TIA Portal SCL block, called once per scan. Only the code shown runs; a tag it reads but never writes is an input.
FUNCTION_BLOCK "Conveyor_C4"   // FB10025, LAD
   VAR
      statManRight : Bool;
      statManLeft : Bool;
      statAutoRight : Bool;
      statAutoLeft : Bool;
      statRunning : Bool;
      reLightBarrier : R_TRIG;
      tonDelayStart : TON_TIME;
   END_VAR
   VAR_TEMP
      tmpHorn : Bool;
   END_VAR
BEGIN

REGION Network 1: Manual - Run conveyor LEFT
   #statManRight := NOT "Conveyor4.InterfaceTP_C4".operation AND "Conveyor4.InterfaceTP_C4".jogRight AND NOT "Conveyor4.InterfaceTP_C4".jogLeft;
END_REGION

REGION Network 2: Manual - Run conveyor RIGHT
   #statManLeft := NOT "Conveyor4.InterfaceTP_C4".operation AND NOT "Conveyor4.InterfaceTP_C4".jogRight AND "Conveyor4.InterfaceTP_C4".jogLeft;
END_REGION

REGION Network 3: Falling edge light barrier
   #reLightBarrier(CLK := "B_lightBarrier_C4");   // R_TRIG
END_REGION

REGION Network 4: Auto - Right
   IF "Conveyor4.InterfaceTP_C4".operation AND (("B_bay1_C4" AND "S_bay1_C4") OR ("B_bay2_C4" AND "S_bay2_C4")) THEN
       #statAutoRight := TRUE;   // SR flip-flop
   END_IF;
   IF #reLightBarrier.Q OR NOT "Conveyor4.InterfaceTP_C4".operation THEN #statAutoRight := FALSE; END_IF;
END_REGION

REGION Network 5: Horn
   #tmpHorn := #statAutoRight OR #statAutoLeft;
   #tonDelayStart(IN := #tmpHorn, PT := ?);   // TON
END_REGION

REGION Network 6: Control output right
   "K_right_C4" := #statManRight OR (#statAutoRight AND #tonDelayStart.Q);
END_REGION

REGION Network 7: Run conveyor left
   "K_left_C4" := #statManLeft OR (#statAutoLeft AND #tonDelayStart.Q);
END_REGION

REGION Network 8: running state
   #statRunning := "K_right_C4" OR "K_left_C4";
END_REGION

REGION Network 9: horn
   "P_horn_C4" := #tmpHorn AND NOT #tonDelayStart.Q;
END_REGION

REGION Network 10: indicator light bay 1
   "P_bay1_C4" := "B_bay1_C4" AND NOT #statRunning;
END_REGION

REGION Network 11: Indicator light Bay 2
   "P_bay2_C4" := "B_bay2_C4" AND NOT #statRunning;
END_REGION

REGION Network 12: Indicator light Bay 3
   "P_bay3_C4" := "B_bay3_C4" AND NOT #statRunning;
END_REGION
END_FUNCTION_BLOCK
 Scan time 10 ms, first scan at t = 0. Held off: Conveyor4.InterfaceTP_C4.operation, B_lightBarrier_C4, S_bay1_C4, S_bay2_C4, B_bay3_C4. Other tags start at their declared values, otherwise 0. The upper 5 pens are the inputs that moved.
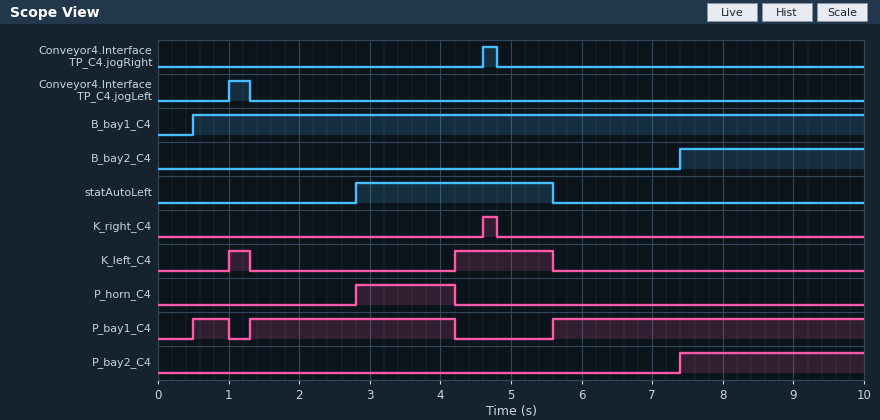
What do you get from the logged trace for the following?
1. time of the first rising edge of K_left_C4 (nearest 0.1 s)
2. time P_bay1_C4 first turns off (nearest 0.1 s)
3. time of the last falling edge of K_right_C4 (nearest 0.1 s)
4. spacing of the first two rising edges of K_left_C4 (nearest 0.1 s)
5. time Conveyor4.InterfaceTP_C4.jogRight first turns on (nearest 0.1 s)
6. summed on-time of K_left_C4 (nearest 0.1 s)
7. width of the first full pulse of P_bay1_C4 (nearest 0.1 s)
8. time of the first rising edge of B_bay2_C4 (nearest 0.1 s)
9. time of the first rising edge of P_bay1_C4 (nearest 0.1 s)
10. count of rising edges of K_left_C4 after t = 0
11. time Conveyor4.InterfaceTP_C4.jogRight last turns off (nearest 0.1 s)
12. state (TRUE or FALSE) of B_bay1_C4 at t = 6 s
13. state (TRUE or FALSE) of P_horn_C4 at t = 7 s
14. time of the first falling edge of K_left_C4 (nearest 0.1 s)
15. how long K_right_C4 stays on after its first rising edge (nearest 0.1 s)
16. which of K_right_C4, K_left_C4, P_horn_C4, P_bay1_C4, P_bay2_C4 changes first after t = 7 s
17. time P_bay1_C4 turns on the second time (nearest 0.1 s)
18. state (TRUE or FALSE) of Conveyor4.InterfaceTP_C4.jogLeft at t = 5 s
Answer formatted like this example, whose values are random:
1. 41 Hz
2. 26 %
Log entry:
1. 1.0 s
2. 1.0 s
3. 4.8 s
4. 3.2 s
5. 4.6 s
6. 1.7 s
7. 0.5 s
8. 7.4 s
9. 0.5 s
10. 2
11. 4.8 s
12. TRUE
13. FALSE
14. 1.3 s
15. 0.2 s
16. P_bay2_C4
17. 1.3 s
18. FALSE
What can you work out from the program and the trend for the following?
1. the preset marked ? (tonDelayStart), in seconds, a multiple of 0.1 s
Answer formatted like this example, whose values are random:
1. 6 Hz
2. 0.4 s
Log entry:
1. 1.4 s
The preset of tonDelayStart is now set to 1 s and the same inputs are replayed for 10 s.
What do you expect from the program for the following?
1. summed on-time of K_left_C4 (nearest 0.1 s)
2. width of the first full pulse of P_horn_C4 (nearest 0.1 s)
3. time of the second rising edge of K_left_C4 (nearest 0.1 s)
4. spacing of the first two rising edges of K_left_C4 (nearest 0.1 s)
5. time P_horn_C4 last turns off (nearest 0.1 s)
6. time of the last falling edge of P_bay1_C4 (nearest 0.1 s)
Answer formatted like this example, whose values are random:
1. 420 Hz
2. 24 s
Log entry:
1. 2.1 s
2. 1.0 s
3. 3.8 s
4. 2.8 s
5. 3.8 s
6. 3.8 s
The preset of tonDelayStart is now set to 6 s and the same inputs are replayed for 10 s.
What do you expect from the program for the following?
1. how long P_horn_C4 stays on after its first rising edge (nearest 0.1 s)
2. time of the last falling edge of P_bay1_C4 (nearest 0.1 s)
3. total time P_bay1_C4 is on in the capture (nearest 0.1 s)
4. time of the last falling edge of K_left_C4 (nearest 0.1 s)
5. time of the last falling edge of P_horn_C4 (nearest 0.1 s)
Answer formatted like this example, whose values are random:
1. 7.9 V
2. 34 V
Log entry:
1. 2.8 s
2. 4.6 s
3. 9.0 s
4. 1.3 s
5. 5.6 s
